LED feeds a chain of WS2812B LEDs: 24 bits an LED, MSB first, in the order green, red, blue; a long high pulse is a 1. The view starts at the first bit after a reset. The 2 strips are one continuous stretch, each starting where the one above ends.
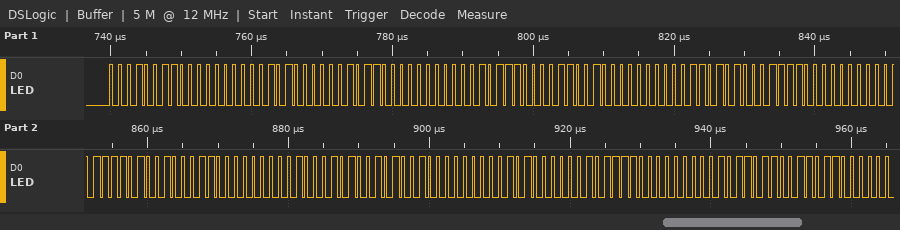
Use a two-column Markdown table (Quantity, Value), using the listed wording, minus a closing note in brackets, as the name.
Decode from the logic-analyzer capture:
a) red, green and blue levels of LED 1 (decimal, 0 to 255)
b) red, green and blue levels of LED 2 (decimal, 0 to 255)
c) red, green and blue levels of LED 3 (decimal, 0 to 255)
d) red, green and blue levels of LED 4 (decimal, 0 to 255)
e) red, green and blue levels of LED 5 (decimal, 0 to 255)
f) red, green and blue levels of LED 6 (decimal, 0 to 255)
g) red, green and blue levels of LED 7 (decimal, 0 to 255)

| Quantity | Value |
|---|---|
| red, green and blue levels of LED 1 | 0, 19, 40 |
| red, green and blue levels of LED 2 | 0, 22, 46 |
| red, green and blue levels of LED 3 | 0, 25, 53 |
| red, green and blue levels of LED 4 | 0, 30, 61 |
| red, green and blue levels of LED 5 | 0, 35, 69 |
| red, green and blue levels of LED 6 | 0, 41, 80 |
| red, green and blue levels of LED 7 | 0, 47, 91 |
